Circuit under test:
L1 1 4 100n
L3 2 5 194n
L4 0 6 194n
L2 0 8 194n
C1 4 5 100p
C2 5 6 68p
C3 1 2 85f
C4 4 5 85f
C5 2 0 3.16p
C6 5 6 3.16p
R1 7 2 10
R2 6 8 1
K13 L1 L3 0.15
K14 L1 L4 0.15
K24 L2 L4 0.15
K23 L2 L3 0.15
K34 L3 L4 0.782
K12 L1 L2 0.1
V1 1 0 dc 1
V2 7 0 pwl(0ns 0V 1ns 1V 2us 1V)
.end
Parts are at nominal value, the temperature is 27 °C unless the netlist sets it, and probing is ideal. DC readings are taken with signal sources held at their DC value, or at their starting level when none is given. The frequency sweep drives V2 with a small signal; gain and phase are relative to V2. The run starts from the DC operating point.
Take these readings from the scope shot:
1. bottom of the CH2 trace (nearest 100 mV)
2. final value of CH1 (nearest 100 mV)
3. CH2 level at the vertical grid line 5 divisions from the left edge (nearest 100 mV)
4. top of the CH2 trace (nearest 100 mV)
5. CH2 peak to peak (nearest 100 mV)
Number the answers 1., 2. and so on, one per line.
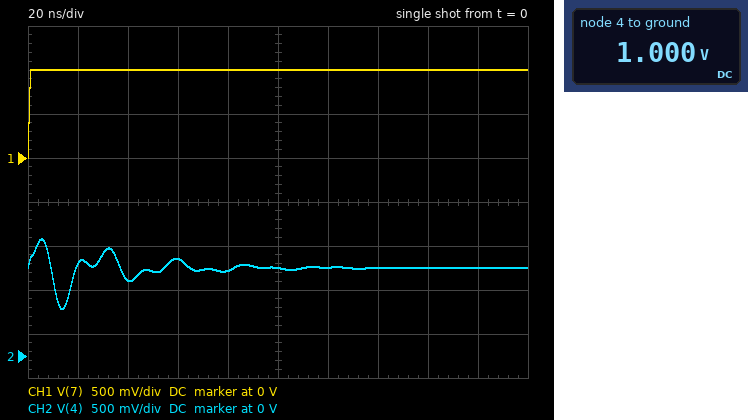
1. 500 mV
2. 1.0 V
3. 1.0 V
4. 1.3 V
5. 800 mV
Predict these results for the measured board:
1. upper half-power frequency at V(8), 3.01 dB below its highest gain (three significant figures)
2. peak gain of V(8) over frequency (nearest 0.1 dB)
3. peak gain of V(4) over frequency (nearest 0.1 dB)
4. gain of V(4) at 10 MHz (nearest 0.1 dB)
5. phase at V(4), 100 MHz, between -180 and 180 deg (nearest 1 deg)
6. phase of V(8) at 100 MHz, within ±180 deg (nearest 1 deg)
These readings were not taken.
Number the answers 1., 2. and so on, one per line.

1. 81.3 MHz
2. 10.6 dB
3. 6.7 dB
4. -29.1 dB
5. -160 deg
6. 20 deg
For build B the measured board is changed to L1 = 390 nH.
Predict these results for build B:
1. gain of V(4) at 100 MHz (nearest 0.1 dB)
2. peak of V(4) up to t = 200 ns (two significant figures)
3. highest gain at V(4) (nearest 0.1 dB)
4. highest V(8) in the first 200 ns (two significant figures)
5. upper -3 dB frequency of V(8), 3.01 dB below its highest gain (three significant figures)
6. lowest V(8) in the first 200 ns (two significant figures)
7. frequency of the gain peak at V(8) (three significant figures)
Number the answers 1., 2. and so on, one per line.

1. -10.3 dB
2. 1.8 V
3. 13.5 dB
4. 220 mV
5. 79.5 MHz
6. -300 mV
7. 70.3 MHz
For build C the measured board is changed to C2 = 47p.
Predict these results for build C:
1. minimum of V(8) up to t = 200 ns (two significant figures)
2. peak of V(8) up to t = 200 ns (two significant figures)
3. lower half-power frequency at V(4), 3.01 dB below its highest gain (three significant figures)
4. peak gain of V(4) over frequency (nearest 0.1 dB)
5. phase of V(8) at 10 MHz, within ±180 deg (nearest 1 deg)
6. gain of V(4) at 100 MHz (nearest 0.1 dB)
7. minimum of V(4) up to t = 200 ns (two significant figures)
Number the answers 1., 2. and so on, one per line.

1. -490 mV
2. 520 mV
3. 82.6 MHz
4. 7.1 dB
5. -4 deg
6. -0.6 dB
7. 560 mV
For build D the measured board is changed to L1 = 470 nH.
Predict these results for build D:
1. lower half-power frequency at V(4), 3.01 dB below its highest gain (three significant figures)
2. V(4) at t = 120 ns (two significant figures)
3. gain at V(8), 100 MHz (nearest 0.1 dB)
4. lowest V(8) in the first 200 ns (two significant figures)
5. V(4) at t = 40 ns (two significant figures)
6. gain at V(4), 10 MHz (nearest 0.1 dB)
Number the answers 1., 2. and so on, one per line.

1. 20.3 MHz
2. 800 mV
3. -5.9 dB
4. -280 mV
5. 1.4 V
6. -13.3 dB
